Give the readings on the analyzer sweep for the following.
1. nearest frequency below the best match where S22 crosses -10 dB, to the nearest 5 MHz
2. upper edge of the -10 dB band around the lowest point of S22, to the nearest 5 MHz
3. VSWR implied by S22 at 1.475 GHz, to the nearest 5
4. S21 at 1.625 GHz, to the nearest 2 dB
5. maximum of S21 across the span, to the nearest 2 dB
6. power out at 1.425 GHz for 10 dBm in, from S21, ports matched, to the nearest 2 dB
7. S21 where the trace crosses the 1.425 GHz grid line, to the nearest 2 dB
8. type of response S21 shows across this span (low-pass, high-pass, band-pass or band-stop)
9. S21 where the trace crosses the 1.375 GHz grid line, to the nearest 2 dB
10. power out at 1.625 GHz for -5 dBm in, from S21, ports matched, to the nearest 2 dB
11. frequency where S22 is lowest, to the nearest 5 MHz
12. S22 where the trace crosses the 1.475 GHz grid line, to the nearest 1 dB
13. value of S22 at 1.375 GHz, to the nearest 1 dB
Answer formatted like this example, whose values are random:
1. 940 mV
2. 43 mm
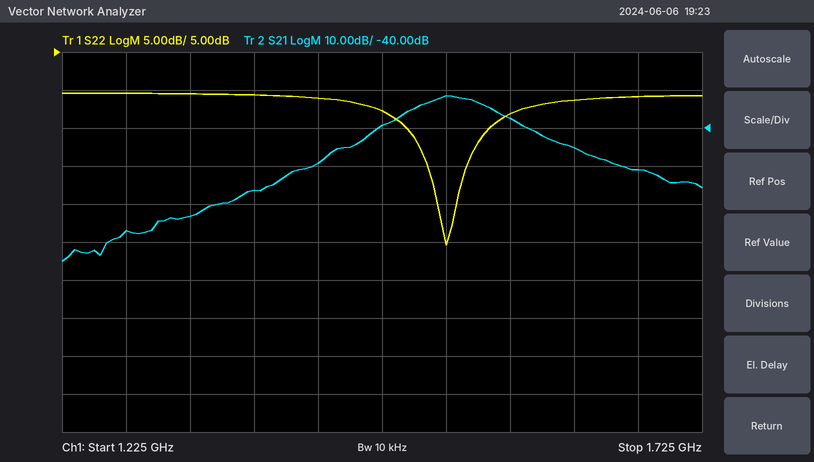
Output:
1. 1.510 GHz
2. 1.540 GHz
3. 5
4. -46 dB
5. -32 dB
6. -40 dBm
7. -50 dB
8. band-pass
9. -56 dB
10. -50 dBm
11. 1.525 GHz
12. -3 dB
13. -1 dB
